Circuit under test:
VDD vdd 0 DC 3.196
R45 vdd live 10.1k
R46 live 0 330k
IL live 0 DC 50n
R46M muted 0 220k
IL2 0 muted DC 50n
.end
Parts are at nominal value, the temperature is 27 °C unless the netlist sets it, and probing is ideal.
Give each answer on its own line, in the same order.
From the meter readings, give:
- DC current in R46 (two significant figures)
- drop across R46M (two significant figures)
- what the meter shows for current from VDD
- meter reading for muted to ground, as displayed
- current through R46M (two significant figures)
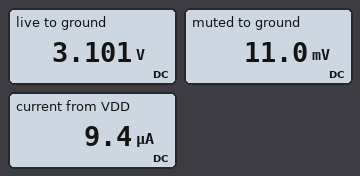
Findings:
9.4 µA
11 mV
9.4 µA
11.0 mV
50 nA
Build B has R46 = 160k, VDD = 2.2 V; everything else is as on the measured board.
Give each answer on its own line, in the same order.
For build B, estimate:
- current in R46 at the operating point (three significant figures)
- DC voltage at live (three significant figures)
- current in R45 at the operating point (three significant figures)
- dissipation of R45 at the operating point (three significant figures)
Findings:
12.9 µA
2.07 V
13.0 µA
1.70 µW
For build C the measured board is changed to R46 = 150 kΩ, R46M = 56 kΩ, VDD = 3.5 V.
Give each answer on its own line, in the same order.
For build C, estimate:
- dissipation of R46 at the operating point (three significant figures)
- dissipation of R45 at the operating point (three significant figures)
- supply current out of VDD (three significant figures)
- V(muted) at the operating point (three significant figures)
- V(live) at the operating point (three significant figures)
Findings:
71.7 µW
4.85 µW
21.9 µA
2.80 mV
3.28 V
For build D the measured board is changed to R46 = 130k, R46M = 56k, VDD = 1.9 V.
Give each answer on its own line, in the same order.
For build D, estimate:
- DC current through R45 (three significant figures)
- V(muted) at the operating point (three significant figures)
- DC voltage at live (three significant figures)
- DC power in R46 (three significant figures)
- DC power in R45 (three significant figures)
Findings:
13.6 µA
2.80 mV
1.76 V
23.9 µW
1.87 µW
